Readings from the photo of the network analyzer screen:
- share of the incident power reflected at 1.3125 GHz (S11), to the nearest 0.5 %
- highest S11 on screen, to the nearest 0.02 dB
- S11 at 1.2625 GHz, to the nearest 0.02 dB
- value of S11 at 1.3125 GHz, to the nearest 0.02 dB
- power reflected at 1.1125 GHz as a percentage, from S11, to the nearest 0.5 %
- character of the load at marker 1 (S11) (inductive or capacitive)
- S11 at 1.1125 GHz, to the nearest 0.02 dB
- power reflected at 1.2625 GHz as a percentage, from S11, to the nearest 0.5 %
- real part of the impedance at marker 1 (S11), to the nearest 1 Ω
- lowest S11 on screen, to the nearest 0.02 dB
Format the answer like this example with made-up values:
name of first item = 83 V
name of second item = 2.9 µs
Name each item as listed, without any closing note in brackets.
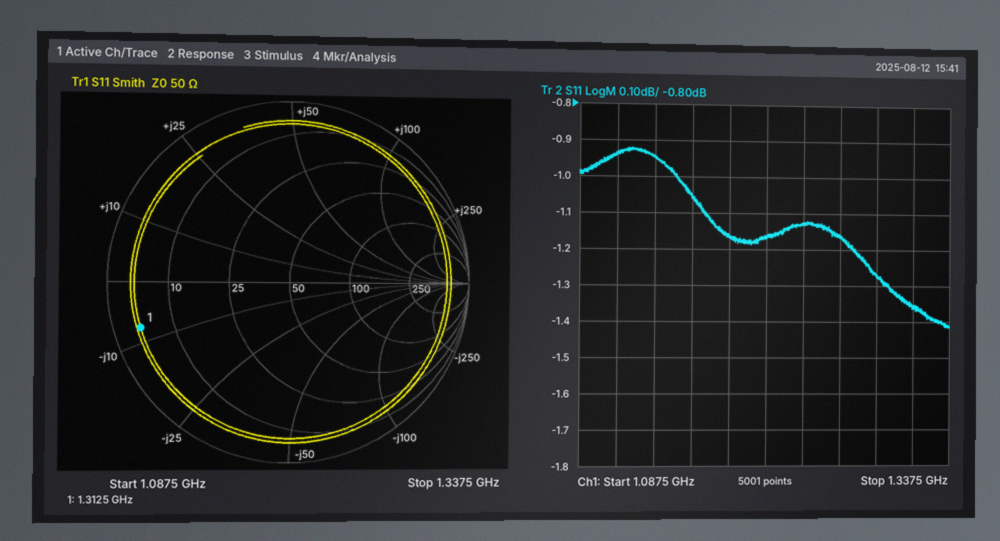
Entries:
share of the incident power reflected at 1.3125 GHz (S11), to the nearest 0.5 % = 73.0 %
highest S11 on screen, to the nearest 0.02 dB = -0.92 dB
S11 at 1.2625 GHz, to the nearest 0.02 dB = -1.16 dB
value of S11 at 1.3125 GHz, to the nearest 0.02 dB = -1.36 dB
power reflected at 1.1125 GHz as a percentage, from S11, to the nearest 0.5 % = 80.5 %
character of the load at marker 1 (S11) = capacitive
S11 at 1.1125 GHz, to the nearest 0.02 dB = -0.94 dB
power reflected at 1.2625 GHz as a percentage, from S11, to the nearest 0.5 % = 76.5 %
real part of the impedance at marker 1 (S11), to the nearest 1 Ω = 4 Ω
lowest S11 on screen, to the nearest 0.02 dB = -1.42 dB
